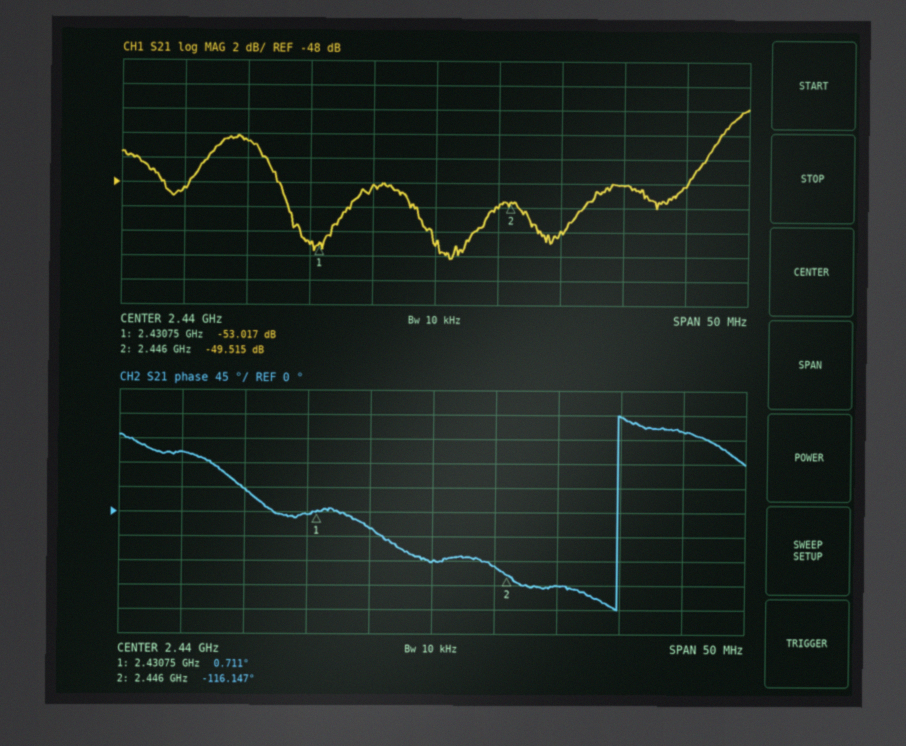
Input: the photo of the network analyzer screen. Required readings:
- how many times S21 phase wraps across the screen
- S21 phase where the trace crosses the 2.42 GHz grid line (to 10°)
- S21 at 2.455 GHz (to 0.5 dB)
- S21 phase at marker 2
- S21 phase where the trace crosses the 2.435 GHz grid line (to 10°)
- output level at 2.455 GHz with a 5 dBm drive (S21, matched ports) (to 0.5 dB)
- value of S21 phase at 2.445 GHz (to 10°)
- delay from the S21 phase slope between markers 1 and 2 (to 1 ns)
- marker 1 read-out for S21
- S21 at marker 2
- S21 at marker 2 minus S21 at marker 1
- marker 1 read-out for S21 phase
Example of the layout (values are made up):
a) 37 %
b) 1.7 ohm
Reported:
a) 1
b) 110°
c) -48.0 dB
d) -116.147°
e) -30°
f) -43.0 dBm
g) -100°
h) 21 ns
i) -53.017 dB
j) -49.515 dB
k) 3.502 dB
l) 0.711°
